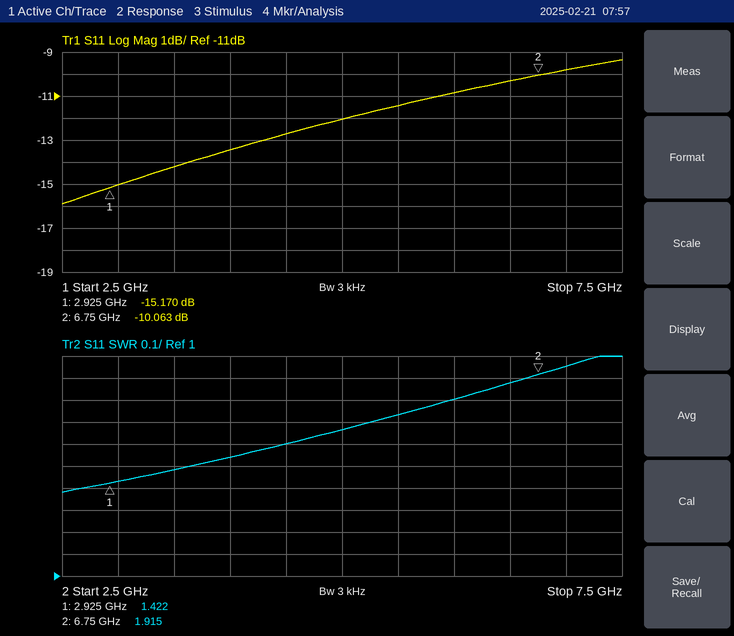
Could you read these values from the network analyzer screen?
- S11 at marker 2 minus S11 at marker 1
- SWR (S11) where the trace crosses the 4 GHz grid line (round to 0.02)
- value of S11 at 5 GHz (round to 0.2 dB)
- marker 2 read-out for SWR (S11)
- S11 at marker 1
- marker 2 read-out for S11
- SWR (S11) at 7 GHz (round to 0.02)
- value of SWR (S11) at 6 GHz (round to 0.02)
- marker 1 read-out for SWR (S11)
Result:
5.107 dB
1.54
-12.0 dB
1.915
-15.170 dB
-10.063 dB
1.96
1.80
1.422
